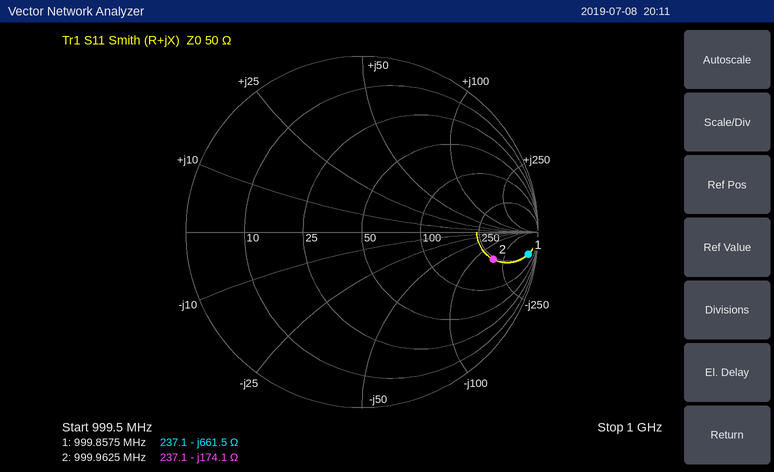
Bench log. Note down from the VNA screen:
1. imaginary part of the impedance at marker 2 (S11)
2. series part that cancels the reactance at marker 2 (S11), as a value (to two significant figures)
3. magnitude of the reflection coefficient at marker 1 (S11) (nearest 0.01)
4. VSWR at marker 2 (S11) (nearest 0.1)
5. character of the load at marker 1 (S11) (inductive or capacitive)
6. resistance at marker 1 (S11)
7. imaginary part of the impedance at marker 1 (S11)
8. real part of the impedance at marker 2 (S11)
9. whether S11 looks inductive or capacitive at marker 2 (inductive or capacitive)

-174.1 Ω
28 nH
0.95
7.4
capacitive
237.1 Ω
-661.5 Ω
237.1 Ω
capacitive
